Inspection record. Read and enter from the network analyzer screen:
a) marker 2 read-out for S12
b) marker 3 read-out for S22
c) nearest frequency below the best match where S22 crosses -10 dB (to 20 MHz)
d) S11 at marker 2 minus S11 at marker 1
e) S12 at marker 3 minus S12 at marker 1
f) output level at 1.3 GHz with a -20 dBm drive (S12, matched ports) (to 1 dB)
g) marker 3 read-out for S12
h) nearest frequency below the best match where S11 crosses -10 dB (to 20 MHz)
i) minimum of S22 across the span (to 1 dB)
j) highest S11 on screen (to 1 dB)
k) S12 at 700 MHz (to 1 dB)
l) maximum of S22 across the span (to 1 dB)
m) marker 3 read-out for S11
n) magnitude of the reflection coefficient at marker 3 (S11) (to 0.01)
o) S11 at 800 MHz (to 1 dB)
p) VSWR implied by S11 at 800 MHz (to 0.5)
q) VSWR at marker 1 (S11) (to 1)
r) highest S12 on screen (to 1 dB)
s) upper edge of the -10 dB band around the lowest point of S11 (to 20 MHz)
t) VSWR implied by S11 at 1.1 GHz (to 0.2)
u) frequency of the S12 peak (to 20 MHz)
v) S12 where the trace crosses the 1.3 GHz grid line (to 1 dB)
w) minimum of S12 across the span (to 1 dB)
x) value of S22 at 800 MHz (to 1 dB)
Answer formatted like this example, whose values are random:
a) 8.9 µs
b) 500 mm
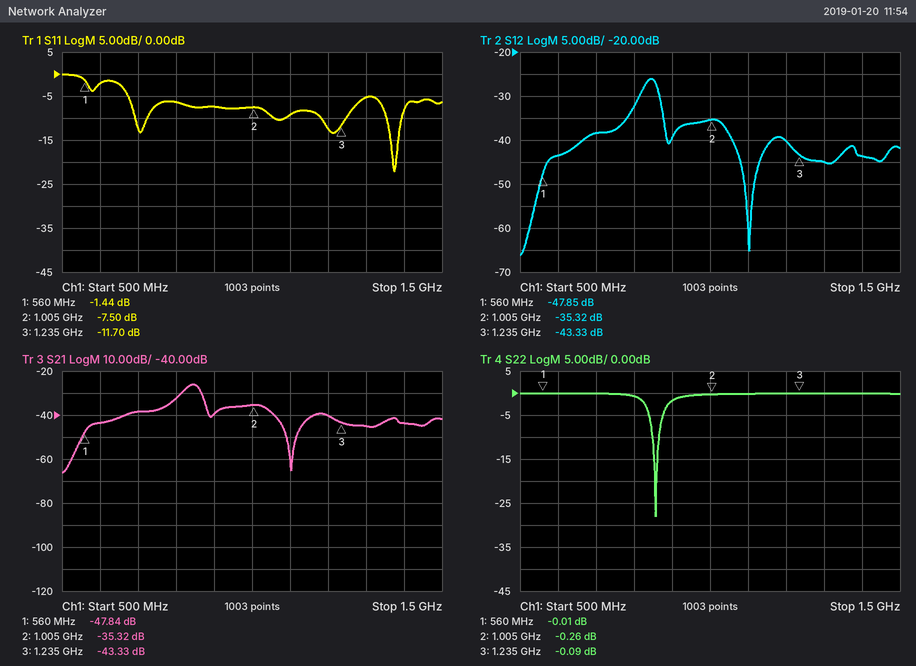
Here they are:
a) -35.32 dB
b) -0.09 dB
c) 840 MHz
d) -6.06 dB
e) 4.52 dB
f) -65 dBm
g) -43.33 dB
h) 1.36 GHz
i) -28 dB
j) 0 dB
k) -38 dB
l) 0 dB
m) -11.70 dB
n) 0.26
o) -6 dB
p) 3.0
q) 12
r) -26 dB
s) 1.40 GHz
t) 2.0
u) 840 MHz
v) -45 dB
w) -66 dB
x) -1 dB
